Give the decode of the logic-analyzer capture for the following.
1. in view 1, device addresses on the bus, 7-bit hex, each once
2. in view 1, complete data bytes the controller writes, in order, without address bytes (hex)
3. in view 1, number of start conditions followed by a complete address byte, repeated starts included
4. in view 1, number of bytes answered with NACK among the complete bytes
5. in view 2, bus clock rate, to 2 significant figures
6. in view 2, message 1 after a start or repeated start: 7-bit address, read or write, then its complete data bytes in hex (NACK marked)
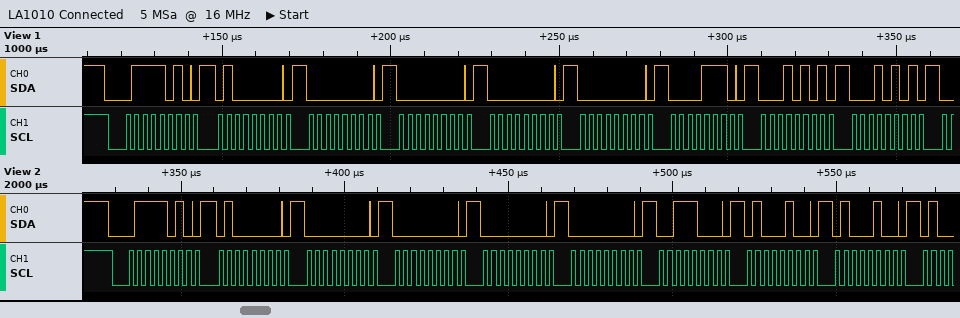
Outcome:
0x3D
40 00 00 00 00 0E 15 15
1
0
400 kHz
0x3D write: 40 00 00 00 00 38 44 44
